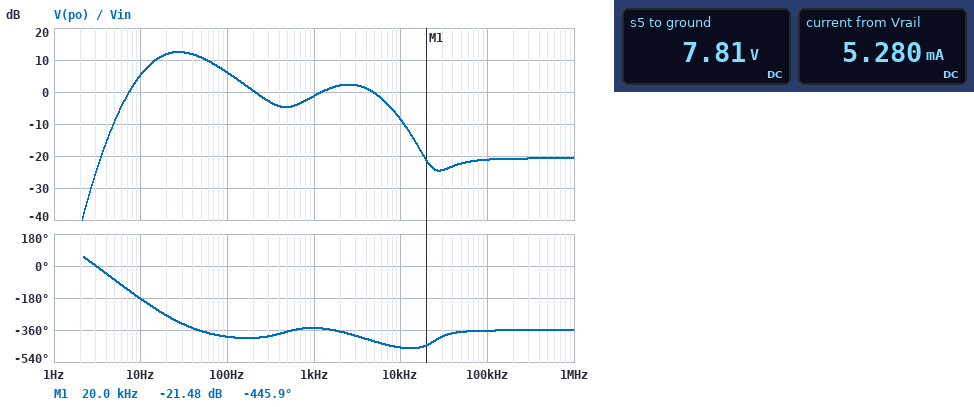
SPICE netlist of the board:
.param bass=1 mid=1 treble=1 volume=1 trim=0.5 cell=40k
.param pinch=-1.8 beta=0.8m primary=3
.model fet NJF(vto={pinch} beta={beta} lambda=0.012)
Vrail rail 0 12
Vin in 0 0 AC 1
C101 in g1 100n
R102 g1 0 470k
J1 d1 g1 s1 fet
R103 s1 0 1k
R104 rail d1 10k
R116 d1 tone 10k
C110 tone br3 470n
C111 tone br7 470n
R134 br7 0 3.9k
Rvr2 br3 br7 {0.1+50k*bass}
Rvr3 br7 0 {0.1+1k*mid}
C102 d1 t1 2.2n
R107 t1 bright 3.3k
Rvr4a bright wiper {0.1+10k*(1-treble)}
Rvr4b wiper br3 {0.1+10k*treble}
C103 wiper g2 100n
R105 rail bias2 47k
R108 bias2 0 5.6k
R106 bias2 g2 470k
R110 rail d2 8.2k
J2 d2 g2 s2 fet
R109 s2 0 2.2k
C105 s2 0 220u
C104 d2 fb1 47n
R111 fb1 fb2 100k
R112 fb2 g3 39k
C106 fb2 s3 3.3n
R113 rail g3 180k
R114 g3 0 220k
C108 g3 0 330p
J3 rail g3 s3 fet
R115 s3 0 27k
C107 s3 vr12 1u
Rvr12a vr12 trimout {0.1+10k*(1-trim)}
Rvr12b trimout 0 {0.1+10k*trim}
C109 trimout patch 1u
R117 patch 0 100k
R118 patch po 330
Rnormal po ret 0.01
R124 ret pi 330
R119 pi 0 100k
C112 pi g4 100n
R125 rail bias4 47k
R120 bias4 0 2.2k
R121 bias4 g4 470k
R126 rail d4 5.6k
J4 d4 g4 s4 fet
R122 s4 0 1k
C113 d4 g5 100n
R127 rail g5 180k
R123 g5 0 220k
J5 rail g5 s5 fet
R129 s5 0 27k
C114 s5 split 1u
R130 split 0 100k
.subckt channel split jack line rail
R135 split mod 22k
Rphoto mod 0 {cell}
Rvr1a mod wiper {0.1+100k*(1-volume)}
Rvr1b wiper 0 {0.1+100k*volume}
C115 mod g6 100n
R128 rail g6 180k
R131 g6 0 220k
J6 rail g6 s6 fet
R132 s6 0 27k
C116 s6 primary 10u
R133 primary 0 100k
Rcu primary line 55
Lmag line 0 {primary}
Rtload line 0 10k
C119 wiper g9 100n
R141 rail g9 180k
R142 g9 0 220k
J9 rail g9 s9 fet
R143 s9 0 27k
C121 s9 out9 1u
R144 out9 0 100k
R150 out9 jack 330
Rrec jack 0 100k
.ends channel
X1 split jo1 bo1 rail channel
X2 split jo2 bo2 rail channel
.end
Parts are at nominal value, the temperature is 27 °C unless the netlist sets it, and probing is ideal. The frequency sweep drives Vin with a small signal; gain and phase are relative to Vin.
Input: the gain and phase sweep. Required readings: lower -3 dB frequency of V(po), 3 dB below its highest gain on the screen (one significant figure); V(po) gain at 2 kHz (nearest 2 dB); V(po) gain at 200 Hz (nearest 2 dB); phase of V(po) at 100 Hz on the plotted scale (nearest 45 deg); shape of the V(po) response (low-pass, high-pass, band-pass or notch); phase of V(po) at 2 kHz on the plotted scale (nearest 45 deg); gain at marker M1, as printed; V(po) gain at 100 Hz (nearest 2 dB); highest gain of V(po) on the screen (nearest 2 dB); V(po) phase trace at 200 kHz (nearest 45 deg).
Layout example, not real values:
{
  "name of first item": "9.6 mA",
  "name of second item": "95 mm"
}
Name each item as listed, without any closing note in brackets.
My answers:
{
  "lower -3 dB frequency of V(po), 3 dB below its highest gain on the screen": "10 Hz",
  "V(po) gain at 2 kHz": "2 dB",
  "V(po) gain at 200 Hz": "0 dB",
  "phase of V(po) at 100 Hz on the plotted scale": "-405 deg",
  "shape of the V(po) response": "band-pass",
  "phase of V(po) at 2 kHz on the plotted scale": "-360 deg",
  "gain at marker M1, as printed": "-21.48 dB",
  "V(po) gain at 100 Hz": "6 dB",
  "highest gain of V(po) on the screen": "12 dB",
  "V(po) phase trace at 200 kHz": "-360 deg"
}
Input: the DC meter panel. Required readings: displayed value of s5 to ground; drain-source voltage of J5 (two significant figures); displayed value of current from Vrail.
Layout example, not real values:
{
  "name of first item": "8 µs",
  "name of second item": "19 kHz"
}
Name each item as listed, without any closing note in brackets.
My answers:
{
  "displayed value of s5 to ground": "7.81 V",
  "drain-source voltage of J5": "4.2 V",
  "displayed value of current from Vrail": "5.280 mA"
}
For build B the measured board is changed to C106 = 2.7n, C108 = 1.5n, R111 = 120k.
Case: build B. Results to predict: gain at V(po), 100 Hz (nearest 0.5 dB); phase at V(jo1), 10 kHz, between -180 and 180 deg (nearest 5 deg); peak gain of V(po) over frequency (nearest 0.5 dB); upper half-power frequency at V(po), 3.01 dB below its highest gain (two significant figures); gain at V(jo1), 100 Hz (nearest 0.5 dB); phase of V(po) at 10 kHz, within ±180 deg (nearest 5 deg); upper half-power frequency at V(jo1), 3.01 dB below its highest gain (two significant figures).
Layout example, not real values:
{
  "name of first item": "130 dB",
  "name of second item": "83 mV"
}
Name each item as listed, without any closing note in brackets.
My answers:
{
  "gain at V(po), 100 Hz": "5.5 dB",
  "phase at V(jo1), 10 kHz, between -180 and 180 deg": "70 deg",
  "peak gain of V(po) over frequency": "12.0 dB",
  "upper half-power frequency at V(po), 3.01 dB below its highest gain": "61 Hz",
  "gain at V(jo1), 100 Hz": "7.5 dB",
  "phase of V(po) at 10 kHz, within ±180 deg": "-110 deg",
  "upper half-power frequency at V(jo1), 3.01 dB below its highest gain": "79 Hz"
}
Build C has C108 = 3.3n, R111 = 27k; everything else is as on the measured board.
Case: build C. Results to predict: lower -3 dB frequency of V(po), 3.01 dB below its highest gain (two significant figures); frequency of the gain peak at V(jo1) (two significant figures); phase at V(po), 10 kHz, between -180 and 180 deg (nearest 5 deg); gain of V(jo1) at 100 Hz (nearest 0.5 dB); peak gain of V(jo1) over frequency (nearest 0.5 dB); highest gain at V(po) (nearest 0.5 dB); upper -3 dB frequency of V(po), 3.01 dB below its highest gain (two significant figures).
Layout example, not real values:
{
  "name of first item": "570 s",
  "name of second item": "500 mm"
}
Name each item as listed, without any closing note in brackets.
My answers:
{
  "lower -3 dB frequency of V(po), 3.01 dB below its highest gain": "15 Hz",
  "frequency of the gain peak at V(jo1)": "39 Hz",
  "phase at V(po), 10 kHz, between -180 and 180 deg": "15 deg",
  "gain of V(jo1) at 100 Hz": "11.0 dB",
  "peak gain of V(jo1) over frequency": "15.0 dB",
  "highest gain at V(po)": "14.5 dB",
  "upper -3 dB frequency of V(po), 3.01 dB below its highest gain": "67 Hz"
}
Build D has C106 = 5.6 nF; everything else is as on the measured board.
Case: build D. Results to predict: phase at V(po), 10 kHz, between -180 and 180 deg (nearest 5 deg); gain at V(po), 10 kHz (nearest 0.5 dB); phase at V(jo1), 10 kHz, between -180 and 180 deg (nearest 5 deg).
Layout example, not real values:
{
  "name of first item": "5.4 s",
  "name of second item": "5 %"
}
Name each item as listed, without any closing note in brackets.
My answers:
{
  "phase at V(po), 10 kHz, between -180 and 180 deg": "-85 deg",
  "gain at V(po), 10 kHz": "-13.5 dB",
  "phase at V(jo1), 10 kHz, between -180 and 180 deg": "95 deg"
}
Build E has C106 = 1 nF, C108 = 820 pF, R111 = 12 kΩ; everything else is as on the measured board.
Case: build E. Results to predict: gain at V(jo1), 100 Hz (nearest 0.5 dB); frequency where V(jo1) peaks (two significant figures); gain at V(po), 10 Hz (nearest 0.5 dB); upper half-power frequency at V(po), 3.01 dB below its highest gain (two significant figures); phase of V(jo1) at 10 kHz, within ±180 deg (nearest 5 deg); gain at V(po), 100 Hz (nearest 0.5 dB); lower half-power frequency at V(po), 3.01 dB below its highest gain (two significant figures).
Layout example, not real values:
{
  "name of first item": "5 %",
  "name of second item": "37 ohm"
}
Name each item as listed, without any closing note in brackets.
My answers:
{
  "gain at V(jo1), 100 Hz": "12.0 dB",
  "frequency where V(jo1) peaks": "40 Hz",
  "gain at V(po), 10 Hz": "6.5 dB",
  "upper half-power frequency at V(po), 3.01 dB below its highest gain": "70 Hz",
  "phase of V(jo1) at 10 kHz, within ±180 deg": "100 deg",
  "gain at V(po), 100 Hz": "10.0 dB",
  "lower half-power frequency at V(po), 3.01 dB below its highest gain": "16 Hz"
}
